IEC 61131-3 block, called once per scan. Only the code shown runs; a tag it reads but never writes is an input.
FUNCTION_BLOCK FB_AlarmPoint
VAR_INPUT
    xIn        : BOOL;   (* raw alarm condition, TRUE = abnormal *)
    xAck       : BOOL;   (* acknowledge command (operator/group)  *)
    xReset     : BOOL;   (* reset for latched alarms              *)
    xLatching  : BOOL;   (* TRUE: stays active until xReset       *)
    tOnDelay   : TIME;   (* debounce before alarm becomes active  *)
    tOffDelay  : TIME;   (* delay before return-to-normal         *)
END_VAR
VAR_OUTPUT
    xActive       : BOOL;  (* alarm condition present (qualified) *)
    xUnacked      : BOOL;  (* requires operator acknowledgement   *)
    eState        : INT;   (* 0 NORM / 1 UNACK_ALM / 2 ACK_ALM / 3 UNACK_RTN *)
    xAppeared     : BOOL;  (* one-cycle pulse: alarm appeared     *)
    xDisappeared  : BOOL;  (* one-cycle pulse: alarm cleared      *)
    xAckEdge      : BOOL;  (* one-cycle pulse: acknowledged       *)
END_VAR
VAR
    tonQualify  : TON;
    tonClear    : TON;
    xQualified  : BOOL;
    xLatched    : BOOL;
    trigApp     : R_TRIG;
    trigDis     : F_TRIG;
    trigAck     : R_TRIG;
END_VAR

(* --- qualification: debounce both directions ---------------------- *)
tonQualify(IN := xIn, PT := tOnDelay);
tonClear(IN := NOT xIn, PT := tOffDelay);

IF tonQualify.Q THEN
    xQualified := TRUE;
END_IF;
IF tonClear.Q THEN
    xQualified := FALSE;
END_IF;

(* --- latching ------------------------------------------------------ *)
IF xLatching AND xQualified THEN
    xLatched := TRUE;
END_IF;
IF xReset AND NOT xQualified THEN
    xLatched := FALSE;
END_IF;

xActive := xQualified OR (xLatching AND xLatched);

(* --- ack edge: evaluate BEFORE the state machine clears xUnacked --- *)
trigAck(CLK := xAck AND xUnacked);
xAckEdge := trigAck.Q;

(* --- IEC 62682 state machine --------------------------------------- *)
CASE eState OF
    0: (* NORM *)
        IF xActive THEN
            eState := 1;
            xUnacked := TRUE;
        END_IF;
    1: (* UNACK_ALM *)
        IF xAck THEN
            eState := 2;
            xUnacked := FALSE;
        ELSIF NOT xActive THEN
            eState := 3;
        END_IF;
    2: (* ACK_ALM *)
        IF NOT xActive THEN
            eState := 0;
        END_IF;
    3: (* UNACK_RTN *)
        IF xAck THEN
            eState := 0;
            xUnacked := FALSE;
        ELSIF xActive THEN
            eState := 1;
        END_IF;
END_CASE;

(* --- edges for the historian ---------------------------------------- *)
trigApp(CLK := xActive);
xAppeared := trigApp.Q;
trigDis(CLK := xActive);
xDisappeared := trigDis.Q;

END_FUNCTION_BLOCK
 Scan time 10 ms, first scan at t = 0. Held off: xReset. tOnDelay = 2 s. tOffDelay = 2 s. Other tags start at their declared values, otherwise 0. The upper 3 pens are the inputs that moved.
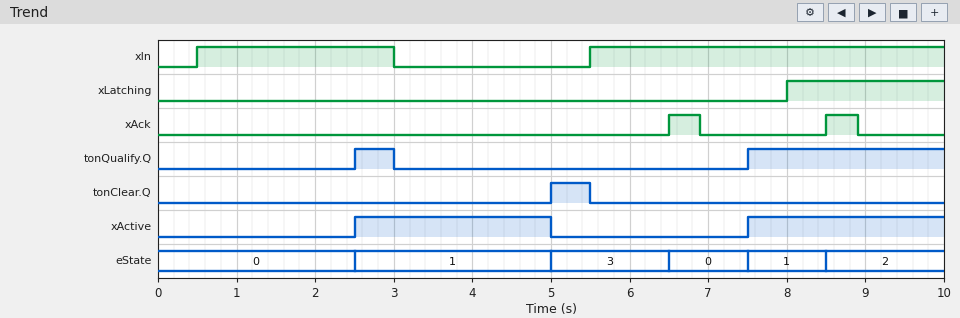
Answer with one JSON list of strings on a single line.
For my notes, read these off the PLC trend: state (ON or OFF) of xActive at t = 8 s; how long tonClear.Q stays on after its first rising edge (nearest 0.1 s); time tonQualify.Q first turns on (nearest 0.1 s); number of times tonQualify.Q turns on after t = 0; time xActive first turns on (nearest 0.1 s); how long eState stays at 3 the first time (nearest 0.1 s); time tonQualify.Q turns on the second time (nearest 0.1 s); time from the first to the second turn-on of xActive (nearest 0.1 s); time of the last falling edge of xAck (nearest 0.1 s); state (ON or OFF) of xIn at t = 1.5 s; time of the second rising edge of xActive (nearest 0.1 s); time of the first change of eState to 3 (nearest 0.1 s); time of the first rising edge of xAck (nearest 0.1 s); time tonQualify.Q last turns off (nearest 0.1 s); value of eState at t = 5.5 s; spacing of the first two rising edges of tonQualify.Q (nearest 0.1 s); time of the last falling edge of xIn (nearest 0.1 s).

["ON", "0.5 s", "2.5 s", "2", "2.5 s", "1.5 s", "7.5 s", "5.0 s", "8.9 s", "ON", "7.5 s", "5.0 s", "6.5 s", "3.0 s", "3", "5.0 s", "3.0 s"]
